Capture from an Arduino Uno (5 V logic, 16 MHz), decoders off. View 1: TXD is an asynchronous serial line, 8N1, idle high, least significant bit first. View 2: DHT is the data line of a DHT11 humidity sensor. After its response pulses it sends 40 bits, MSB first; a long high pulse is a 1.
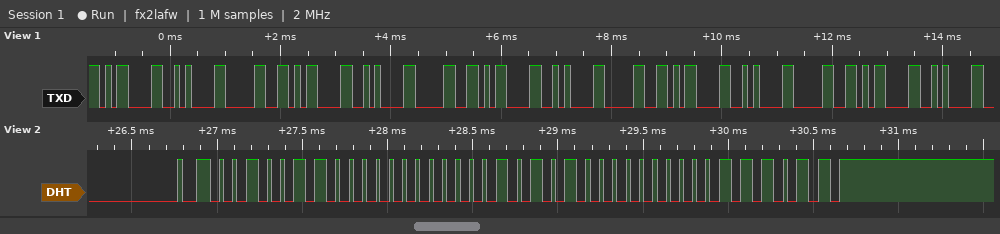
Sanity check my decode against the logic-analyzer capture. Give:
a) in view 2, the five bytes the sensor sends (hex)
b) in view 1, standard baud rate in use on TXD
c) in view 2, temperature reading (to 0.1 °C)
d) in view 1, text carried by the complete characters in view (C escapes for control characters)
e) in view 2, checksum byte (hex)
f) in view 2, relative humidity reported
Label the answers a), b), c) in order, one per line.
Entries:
a) 26 00 15 00 3B
b) 9600 baud
c) 21.0 °C
d) "\r\n0\r\n0\r\n0\r\n0\r\n"
e) 0x3B
f) 38 %
